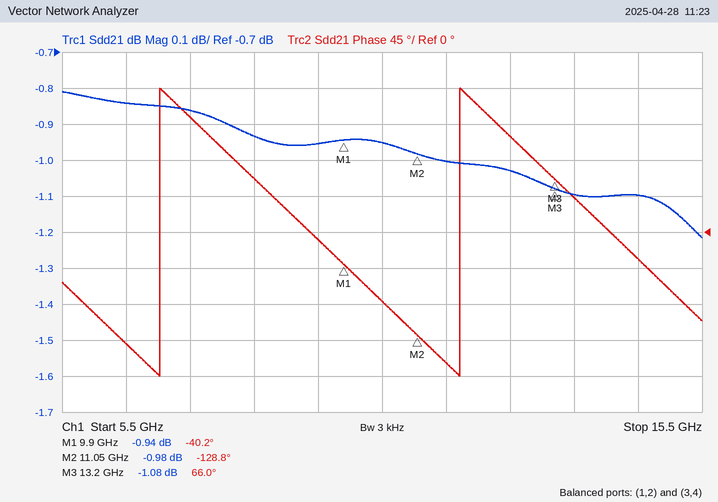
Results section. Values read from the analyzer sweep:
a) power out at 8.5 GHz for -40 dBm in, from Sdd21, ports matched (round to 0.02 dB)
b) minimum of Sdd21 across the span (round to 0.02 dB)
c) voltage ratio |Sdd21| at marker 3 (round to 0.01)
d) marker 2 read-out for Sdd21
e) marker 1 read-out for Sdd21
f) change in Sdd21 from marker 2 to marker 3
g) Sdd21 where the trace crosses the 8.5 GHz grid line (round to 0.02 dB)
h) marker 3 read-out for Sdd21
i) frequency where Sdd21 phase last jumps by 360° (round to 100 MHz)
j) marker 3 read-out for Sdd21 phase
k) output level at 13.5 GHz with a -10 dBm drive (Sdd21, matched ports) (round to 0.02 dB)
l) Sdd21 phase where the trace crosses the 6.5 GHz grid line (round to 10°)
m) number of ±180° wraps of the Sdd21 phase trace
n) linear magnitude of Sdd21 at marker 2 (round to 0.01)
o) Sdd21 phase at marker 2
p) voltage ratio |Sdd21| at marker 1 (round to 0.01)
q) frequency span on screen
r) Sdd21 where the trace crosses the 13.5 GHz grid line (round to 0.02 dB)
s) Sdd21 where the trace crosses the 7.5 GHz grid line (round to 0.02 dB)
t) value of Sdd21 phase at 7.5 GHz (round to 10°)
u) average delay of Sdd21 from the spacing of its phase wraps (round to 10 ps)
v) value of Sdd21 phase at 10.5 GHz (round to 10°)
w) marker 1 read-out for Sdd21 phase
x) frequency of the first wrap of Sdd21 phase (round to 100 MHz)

-40.94 dBm
-1.22 dB
0.88
-0.98 dB
-0.94 dB
-0.10 dB
-0.94 dB
-1.08 dB
11.7 GHz
66.0°
-11.10 dBm
-140°
2
0.89
-128.8°
0.90
10 GHz
-1.10 dB
-0.86 dB
140°
210 ps
-90°
-40.2°
7.0 GHz
